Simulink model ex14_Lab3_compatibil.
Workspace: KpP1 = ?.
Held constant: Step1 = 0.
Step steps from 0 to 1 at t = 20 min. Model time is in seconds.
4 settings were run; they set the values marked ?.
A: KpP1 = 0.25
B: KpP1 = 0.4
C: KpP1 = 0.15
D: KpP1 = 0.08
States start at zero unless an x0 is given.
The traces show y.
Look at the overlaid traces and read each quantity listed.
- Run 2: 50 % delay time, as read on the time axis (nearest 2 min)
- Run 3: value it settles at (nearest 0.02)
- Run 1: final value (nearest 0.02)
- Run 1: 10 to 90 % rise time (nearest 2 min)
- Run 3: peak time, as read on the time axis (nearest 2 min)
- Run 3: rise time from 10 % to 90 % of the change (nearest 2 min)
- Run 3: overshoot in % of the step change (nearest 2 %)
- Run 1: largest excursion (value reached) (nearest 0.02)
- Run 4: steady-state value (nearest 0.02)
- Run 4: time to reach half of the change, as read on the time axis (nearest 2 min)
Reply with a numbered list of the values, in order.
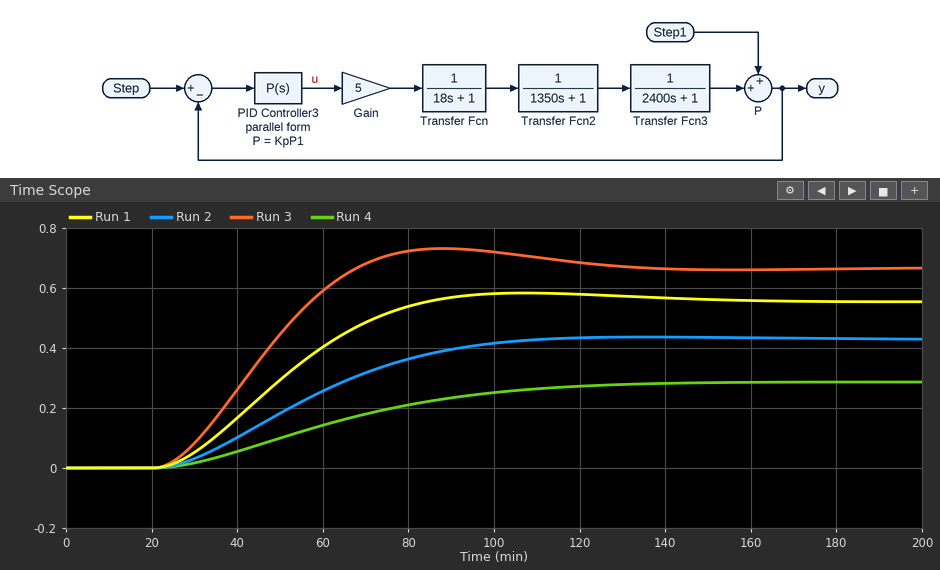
1. 54 min
2. 0.66
3. 0.56
4. 42 min
5. 88 min
6. 32 min
7. 10 %
8. 0.58
9. 0.28
10. 60 min
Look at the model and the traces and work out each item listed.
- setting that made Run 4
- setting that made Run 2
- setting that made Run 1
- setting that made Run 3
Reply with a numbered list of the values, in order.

1. D
2. C
3. A
4. B
